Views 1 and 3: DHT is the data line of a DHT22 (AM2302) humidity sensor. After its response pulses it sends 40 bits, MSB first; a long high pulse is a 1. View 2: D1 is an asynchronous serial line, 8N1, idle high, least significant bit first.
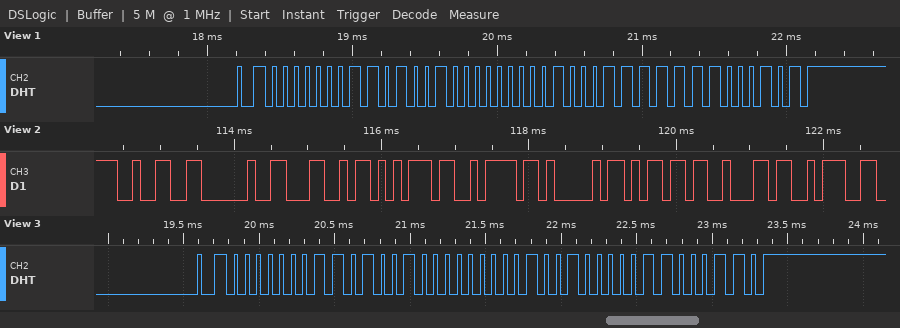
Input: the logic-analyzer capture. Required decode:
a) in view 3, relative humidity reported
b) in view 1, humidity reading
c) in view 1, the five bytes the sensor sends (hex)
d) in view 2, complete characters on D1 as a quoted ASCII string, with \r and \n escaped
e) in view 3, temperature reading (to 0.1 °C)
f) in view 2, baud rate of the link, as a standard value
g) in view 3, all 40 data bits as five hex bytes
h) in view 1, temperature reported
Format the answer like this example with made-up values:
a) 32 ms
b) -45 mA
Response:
a) 42.0 %
b) 42.0 %
c) 01 A4 01 1F C5
d) "2 LuzAmb:"
e) 28.8 °C
f) 9600 baud
g) 01 A4 01 20 C6
h) 28.7 °C
